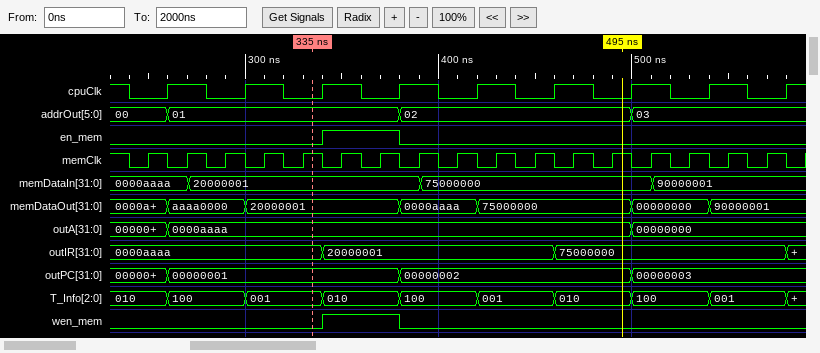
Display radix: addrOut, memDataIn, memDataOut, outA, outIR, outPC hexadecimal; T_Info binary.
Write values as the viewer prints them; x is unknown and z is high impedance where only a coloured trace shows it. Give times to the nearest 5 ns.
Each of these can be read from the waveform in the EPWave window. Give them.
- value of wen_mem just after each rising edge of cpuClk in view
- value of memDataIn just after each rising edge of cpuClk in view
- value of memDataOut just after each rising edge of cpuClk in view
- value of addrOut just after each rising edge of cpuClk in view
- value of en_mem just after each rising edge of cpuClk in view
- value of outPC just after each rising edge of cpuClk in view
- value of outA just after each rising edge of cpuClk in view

0 0 1 0 0 0 0 0 0
0000aaaa, 20000001, 20000001, 20000001, 75000000, 75000000, 75000000, 90000001, 90000001
aaaa0000, 20000001, 20000001, 0000aaaa, 75000000, 75000000, 00000000, 90000001, 90000001
01, 01, 01, 02, 02, 02, 03, 03, 03
0 0 1 0 0 0 0 0 0
00000001, 00000001, 00000001, 00000002, 00000002, 00000002, 00000003, 00000003, 00000003
0000aaaa, 0000aaaa, 0000aaaa, 0000aaaa, 0000aaaa, 0000aaaa, 00000000, 00000000, 00000000
